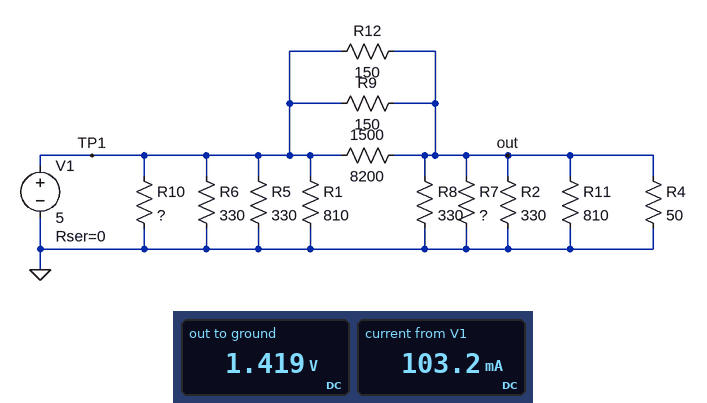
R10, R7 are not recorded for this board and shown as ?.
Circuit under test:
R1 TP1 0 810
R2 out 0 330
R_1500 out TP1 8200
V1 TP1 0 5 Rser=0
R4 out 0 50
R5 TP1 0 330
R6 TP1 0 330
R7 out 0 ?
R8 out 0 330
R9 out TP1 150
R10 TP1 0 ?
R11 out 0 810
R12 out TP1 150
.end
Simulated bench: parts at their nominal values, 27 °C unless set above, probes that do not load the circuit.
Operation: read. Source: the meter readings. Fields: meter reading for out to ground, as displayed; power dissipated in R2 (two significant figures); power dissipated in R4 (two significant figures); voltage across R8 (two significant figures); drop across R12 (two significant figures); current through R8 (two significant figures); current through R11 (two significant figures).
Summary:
1.419 V
6.1 mW
40 mW
1.4 V
3.6 V
4.3 mA
1.8 mA
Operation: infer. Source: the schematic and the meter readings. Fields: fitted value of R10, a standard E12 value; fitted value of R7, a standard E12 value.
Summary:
270 Ω
150 Ω
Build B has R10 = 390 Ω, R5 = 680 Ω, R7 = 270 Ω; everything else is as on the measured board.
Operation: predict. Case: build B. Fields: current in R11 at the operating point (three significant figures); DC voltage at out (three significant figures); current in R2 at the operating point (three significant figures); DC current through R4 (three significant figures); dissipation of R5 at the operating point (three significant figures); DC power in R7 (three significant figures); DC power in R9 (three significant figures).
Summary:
1.87 mA
1.51 V
4.59 mA
30.3 mA
36.8 mW
8.48 mW
81.0 mW
